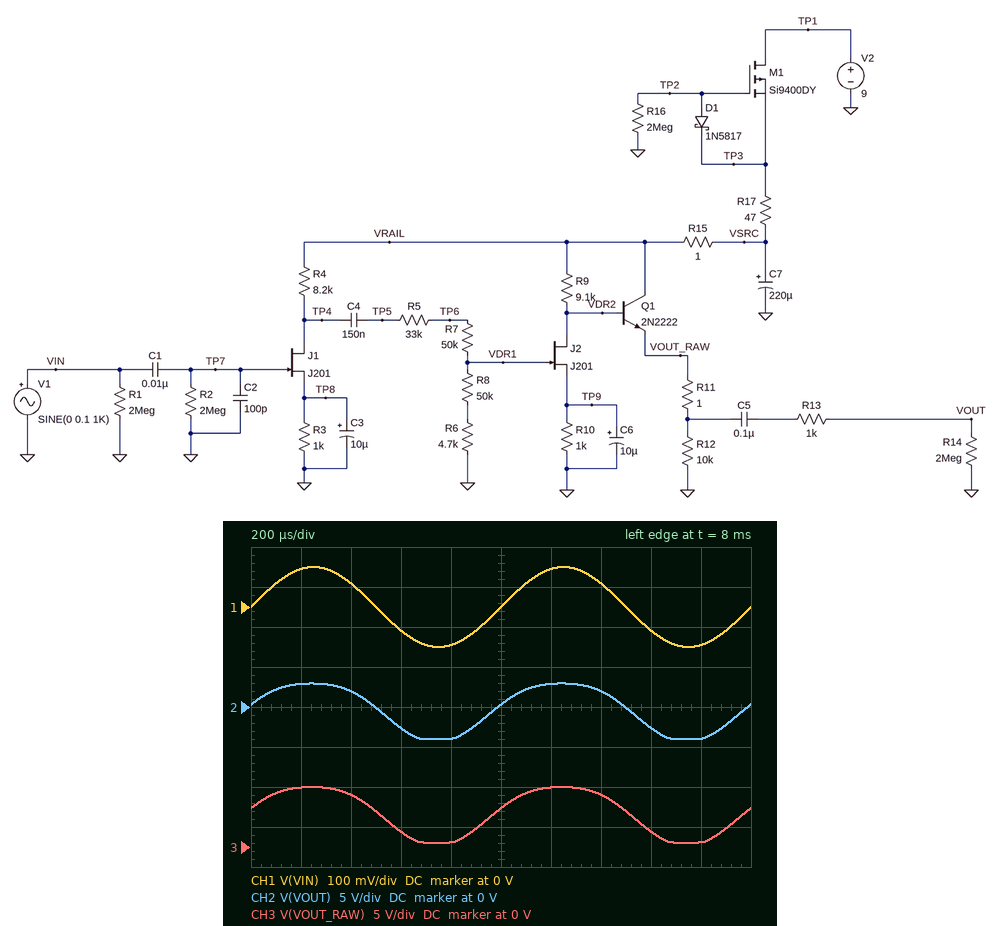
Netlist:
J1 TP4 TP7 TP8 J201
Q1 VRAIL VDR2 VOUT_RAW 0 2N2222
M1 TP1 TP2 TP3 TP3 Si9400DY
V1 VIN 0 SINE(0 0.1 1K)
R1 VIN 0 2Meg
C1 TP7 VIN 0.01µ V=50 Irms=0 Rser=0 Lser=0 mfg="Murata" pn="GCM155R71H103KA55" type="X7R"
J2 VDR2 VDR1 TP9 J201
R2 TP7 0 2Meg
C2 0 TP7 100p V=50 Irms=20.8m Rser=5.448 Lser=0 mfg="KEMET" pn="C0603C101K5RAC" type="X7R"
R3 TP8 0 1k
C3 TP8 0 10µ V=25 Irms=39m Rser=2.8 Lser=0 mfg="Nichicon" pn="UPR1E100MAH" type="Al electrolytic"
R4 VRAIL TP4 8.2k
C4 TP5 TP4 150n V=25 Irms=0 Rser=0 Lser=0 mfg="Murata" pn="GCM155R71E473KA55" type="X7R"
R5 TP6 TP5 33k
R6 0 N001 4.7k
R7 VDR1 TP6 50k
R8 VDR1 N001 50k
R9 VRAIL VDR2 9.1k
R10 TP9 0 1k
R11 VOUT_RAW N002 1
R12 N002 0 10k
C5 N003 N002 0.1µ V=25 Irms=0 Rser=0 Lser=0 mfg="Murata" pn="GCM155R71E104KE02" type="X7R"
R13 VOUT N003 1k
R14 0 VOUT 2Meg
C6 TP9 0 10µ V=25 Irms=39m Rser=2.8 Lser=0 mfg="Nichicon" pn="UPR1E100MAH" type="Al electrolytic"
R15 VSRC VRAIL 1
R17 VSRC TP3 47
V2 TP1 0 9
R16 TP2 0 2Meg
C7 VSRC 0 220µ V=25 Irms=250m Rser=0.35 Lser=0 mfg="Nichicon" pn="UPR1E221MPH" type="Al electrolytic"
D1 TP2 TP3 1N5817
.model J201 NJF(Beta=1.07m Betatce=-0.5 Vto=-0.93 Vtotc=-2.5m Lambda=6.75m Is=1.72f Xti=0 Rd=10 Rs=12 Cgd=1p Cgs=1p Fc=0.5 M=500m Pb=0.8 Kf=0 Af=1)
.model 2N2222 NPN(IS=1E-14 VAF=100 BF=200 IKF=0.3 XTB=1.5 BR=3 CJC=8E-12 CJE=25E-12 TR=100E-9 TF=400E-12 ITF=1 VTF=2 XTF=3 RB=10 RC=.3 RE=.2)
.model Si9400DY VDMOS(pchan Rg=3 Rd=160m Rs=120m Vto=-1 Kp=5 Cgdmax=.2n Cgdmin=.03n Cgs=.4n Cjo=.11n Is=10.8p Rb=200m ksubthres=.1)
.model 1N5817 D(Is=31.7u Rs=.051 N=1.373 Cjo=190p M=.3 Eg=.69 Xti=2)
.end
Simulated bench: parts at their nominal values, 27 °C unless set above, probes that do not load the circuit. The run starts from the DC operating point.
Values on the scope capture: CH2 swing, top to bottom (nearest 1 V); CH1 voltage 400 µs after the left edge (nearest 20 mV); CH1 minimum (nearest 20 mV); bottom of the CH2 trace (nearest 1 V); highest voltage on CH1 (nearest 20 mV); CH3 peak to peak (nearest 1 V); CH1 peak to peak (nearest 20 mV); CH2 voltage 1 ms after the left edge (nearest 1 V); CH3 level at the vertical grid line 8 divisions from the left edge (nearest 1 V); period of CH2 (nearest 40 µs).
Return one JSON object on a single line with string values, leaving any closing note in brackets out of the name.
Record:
{"CH2 swing, top to bottom": "7 V", "CH1 voltage 400 µs after the left edge": "60 mV", "CH1 minimum": "-100 mV", "bottom of the CH2 trace": "-4 V", "highest voltage on CH1": "100 mV", "CH3 peak to peak": "7 V", "CH1 peak to peak": "200 mV", "CH2 voltage 1 ms after the left edge": "0 V", "CH3 level at the vertical grid line 8 divisions from the left edge": "2 V", "period of CH2": "1.00 ms"}
